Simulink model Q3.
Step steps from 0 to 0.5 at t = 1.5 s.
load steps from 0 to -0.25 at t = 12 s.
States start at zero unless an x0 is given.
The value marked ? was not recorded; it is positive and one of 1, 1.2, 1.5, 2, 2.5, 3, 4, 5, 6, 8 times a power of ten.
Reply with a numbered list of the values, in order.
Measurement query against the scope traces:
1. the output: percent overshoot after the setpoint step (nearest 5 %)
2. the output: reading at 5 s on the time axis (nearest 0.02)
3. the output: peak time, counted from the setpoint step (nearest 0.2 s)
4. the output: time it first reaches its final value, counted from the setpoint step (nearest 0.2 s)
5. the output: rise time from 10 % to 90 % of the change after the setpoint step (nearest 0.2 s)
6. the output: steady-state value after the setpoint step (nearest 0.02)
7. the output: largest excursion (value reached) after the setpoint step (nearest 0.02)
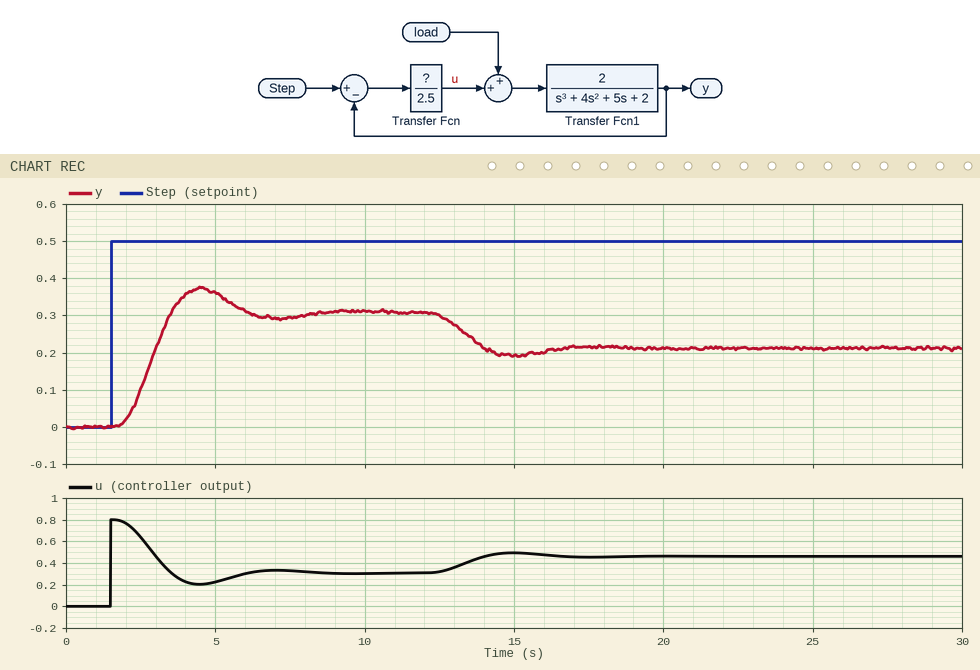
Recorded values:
1. 20 %
2. 0.36
3. 3.0 s
4. 2.0 s
5. 1.2 s
6. 0.30
7. 0.38
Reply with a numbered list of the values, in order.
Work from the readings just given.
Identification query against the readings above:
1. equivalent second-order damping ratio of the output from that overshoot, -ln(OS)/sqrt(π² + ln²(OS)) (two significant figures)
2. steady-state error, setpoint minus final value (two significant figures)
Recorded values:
1. 0.46
2. 0.20
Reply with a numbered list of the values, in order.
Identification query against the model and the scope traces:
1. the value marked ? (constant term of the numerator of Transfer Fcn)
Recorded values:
1. 4
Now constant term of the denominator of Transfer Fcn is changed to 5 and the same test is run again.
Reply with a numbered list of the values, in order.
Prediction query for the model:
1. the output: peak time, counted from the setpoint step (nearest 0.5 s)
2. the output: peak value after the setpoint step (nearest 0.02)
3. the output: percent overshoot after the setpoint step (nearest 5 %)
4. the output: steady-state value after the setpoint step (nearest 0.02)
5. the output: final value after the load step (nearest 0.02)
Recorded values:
1. 4.0 s
2. 0.24
3. 10 %
4. 0.22
5. 0.08
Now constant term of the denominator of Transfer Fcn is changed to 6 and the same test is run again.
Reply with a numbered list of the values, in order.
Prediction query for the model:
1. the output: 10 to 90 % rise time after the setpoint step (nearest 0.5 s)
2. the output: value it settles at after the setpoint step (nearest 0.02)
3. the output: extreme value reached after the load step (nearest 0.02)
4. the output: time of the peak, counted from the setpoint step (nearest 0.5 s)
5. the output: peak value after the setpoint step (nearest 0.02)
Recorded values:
1. 2.0 s
2. 0.20
3. 0.04
4. 4.0 s
5. 0.22
